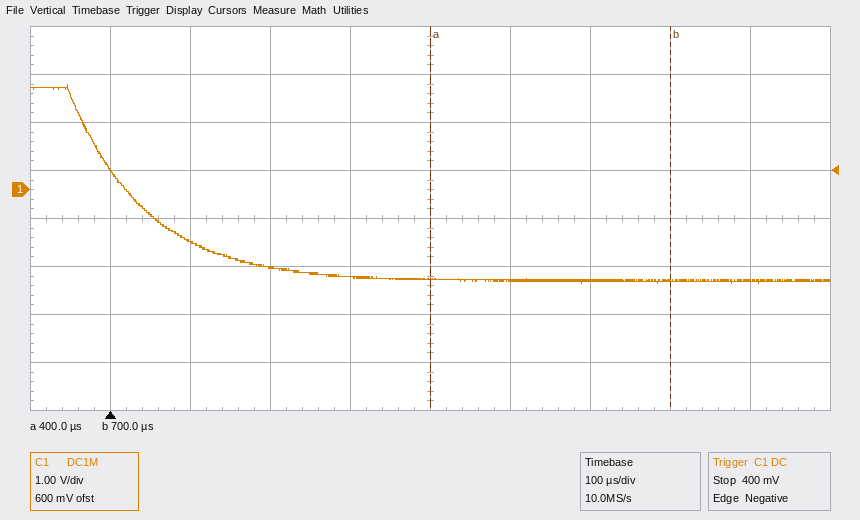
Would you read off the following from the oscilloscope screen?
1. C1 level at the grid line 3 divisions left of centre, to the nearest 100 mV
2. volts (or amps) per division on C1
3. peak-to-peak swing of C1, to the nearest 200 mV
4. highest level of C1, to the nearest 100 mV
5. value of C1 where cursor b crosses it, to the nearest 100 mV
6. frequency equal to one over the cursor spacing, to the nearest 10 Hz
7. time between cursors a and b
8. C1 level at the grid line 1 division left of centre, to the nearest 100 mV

-1.1 V
1 V
4.2 V
2.2 V
-1.9 V
3.33 kHz
300 µs
-1.8 V
